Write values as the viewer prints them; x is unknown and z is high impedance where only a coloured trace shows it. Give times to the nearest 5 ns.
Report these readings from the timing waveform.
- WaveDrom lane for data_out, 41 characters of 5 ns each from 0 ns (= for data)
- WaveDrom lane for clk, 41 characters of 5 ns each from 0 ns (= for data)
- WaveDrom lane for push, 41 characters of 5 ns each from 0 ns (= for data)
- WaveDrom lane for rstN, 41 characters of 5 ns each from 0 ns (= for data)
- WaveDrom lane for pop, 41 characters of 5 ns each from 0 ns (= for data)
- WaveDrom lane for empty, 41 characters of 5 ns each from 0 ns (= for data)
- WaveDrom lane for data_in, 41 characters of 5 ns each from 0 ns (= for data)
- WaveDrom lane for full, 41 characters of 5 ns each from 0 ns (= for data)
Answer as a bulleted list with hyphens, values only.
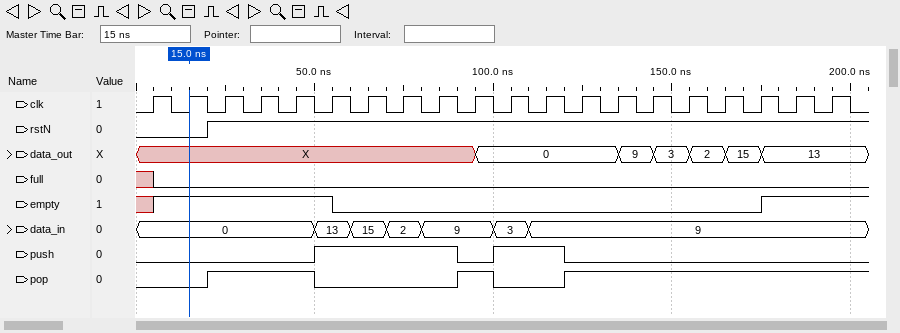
- {name: 'data_out', wave: 'x..................=.......=.=.=.=.=.....', data: '0 9 3 2 15 13'}
- {name: 'clk', wave: '01010101010101010101010101010101010101010'}
- {name: 'push', wave: '0.........1.......0.1...0................'}
- {name: 'rstN', wave: '0...1....................................'}
- {name: 'pop', wave: '0...1.....0.......1.0...1................'}
- {name: 'empty', wave: 'x1.........0.......................1.....'}
- {name: 'data_in', wave: '=.........=.=.=.=...=.=..................', data: '0 13 15 2 9 3 9'}
- {name: 'full', wave: 'x0.......................................'}
